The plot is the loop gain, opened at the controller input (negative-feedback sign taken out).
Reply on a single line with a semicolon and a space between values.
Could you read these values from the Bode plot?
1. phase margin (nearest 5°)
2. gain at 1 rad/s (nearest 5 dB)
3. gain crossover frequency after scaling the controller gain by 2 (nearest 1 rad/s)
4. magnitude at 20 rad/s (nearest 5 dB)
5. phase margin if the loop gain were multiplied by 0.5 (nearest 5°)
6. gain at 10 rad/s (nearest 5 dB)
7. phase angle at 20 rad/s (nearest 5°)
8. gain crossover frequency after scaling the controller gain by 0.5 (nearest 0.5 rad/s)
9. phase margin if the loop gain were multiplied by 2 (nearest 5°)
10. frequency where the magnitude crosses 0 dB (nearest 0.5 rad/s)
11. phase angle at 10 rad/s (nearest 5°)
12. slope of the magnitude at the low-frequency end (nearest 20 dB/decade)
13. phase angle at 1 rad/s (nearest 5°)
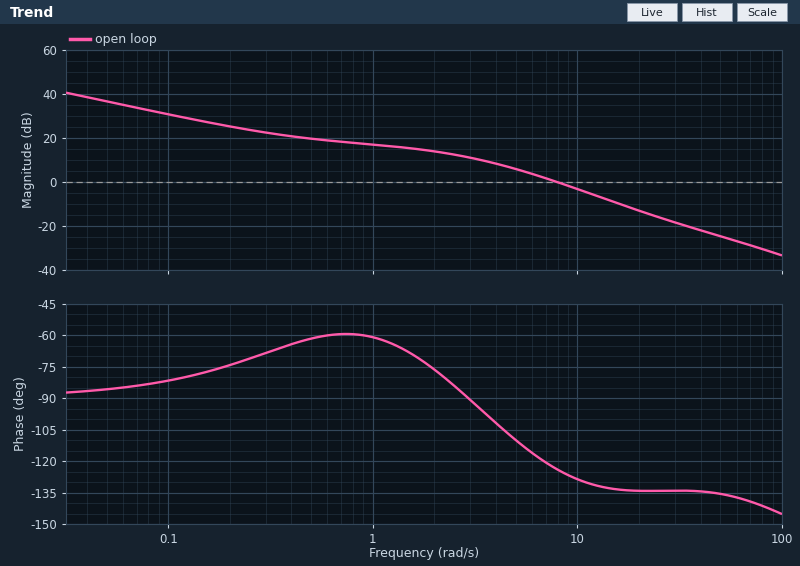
55°; 15 dB; 12 rad/s; -15 dB; 70°; -5 dB; -135°; 5.0 rad/s; 50°; 8.0 rad/s; -130°; -20 dB/decade; -60°
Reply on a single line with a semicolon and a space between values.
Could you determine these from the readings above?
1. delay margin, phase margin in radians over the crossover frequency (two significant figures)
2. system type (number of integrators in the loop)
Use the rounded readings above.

0.12 s; 1
